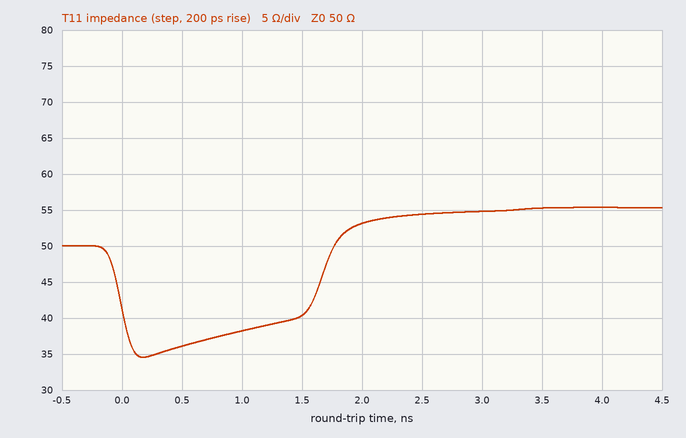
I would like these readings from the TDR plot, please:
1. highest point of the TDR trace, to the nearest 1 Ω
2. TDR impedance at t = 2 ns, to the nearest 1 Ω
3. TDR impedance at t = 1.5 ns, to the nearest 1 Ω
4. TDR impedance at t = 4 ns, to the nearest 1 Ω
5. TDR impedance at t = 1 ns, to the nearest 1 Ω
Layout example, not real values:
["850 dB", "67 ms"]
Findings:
["55 Ω", "53 Ω", "40 Ω", "55 Ω", "38 Ω"]
